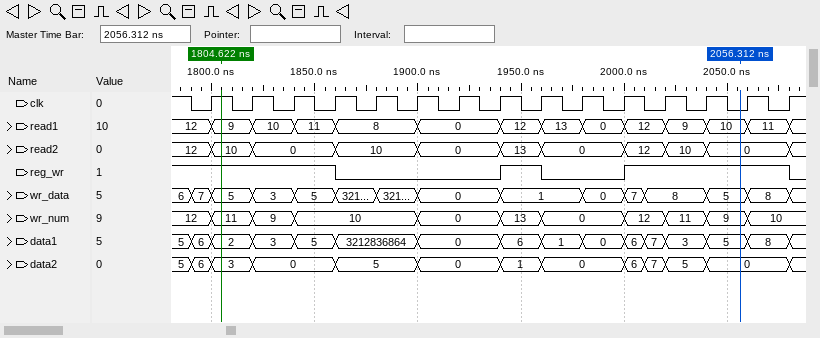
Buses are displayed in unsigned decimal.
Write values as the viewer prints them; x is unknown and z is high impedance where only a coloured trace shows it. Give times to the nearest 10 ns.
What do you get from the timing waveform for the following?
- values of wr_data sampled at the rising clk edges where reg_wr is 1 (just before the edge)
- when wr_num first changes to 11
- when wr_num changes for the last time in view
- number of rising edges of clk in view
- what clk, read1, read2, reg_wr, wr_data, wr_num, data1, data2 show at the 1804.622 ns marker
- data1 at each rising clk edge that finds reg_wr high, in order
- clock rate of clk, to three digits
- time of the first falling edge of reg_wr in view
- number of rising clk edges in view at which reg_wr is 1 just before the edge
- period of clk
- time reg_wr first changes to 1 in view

7, 5, 3, 5, 1, 8, 8, 5, 8
1800 ns
2060 ns
15
clk=1, read1=9, read2=10, reg_wr=1, wr_data=5, wr_num=11, data1=2, data2=3
6, 2, 3, 5, 6, 7, 3, 5, 8
50.0 MHz
1860 ns
9
20 ns
1940 ns
